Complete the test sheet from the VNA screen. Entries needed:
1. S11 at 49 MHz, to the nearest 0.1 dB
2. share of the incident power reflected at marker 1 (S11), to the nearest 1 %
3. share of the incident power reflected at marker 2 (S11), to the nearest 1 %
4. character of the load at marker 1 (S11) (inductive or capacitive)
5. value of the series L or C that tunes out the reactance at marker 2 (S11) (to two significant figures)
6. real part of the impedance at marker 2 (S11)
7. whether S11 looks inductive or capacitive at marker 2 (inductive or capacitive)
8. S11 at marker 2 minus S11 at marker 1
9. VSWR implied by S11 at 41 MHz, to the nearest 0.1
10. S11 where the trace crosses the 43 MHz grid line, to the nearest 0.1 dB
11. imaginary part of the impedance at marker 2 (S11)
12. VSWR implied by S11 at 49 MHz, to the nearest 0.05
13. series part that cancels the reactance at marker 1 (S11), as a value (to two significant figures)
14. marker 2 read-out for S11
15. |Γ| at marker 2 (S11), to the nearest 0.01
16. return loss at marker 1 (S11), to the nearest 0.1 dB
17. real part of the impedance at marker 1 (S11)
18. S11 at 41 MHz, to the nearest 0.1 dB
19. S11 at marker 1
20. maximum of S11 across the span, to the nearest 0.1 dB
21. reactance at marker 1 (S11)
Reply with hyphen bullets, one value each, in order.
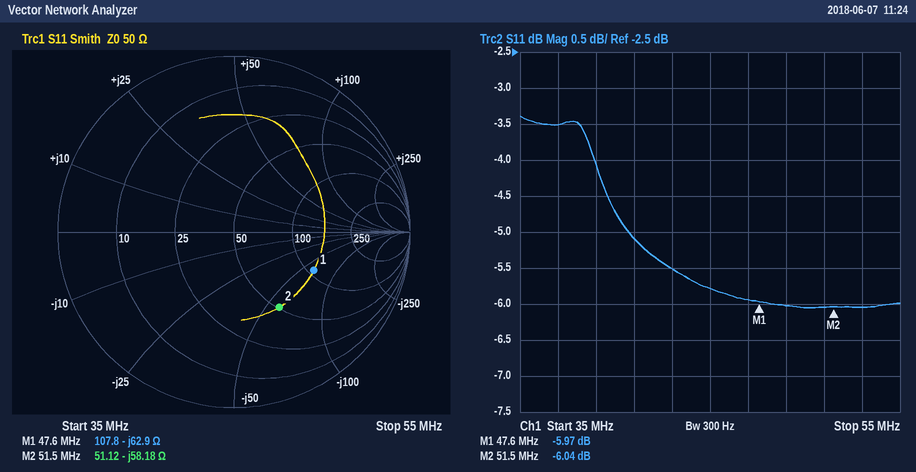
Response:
- -6.0 dB
- 25 %
- 25 %
- capacitive
- 180 nH
- 51.12 Ω
- capacitive
- -0.07 dB
- 3.5
- -5.5 dB
- -58.18 Ω
- 3.00
- 210 nH
- -6.04 dB
- 0.50
- 6.0 dB
- 107.8 Ω
- -5.1 dB
- -5.97 dB
- -3.4 dB
- -62.9 Ω
